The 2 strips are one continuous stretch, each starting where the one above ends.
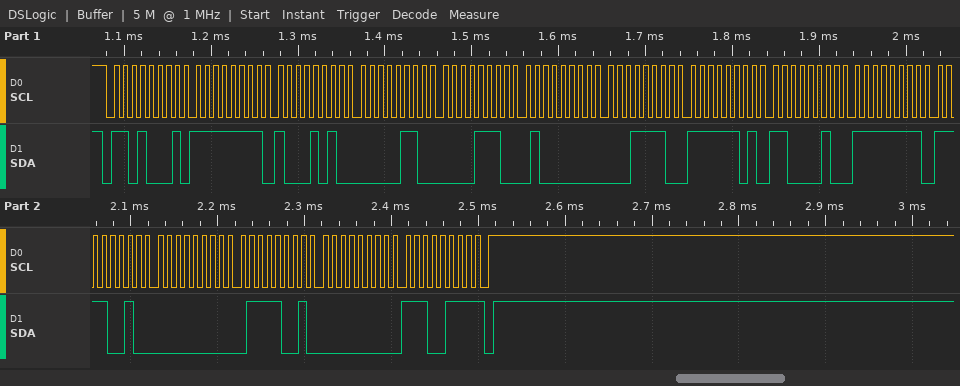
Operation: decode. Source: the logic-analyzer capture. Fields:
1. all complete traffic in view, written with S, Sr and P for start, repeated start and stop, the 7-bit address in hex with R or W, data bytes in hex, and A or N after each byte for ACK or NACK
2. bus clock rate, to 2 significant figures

S 68R A FF A 8A A 06 A 0E A 40 A 1E A FD A C2 A FF A F2 A 00 A 79 A 00 A E7 N P
100 kHz
